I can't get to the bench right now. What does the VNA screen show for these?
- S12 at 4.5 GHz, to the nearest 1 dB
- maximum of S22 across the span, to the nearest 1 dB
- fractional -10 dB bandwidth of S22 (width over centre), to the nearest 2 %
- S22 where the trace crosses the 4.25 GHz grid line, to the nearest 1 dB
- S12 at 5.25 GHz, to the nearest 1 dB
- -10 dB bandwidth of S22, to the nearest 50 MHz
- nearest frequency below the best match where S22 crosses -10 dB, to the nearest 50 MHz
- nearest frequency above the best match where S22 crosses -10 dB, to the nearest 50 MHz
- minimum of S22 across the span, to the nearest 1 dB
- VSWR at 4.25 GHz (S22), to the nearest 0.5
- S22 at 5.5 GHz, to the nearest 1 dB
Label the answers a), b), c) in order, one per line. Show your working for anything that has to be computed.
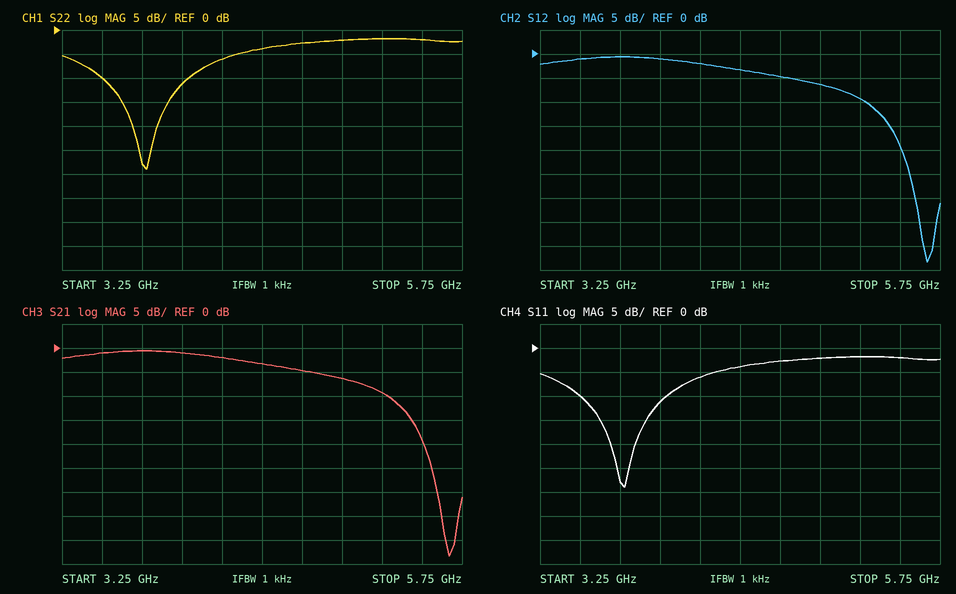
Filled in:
a) -3 dB
b) -2 dB
c) 550 MHz / 3.775 GHz ≈ 14.6 %, so 14 % to the nearest 2 %
d) -6 dB
e) -9 dB
f) 4.05 GHz − 3.50 GHz = 550 MHz
g) 3.50 GHz
h) 4.05 GHz
i) -29 dB
j) |Γ| = 10^(-6/20) = 0.5012; VSWR = (1 + 0.5012)/(1 − 0.5012) ≈ 3.0
k) -2 dB
